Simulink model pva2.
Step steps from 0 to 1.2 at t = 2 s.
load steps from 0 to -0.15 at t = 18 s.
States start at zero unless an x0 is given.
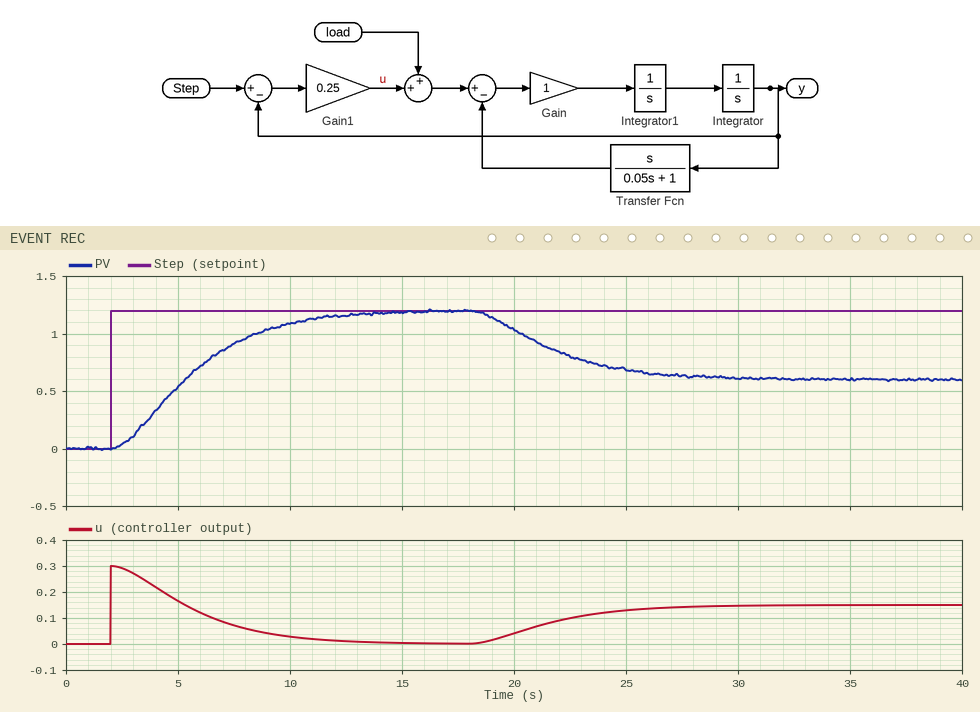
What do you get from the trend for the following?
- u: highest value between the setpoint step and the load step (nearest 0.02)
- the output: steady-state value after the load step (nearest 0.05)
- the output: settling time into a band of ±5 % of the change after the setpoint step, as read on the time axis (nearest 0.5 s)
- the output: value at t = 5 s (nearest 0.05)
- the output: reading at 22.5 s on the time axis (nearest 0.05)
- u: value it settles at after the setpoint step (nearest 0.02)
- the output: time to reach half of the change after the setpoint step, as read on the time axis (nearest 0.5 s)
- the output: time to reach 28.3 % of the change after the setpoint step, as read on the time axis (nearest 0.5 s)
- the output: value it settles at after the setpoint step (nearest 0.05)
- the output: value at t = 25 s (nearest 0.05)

0.30
0.60
11.5 s
0.55
0.80
0.00
5.5 s
4.0 s
1.20
0.70
